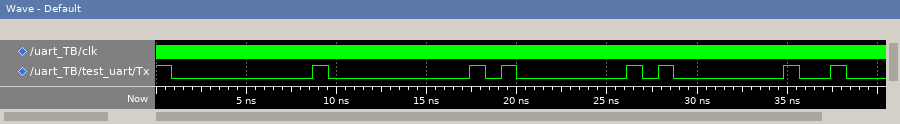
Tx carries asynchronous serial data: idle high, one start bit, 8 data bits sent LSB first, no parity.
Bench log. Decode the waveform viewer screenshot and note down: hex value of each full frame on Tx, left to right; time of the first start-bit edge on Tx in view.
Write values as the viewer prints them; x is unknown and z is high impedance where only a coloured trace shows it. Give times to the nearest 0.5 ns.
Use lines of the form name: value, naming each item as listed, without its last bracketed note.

hex value of each full frame on Tx, left to right: 00, 00, 01, 01
time of the first start-bit edge on Tx in view: 1 ns
